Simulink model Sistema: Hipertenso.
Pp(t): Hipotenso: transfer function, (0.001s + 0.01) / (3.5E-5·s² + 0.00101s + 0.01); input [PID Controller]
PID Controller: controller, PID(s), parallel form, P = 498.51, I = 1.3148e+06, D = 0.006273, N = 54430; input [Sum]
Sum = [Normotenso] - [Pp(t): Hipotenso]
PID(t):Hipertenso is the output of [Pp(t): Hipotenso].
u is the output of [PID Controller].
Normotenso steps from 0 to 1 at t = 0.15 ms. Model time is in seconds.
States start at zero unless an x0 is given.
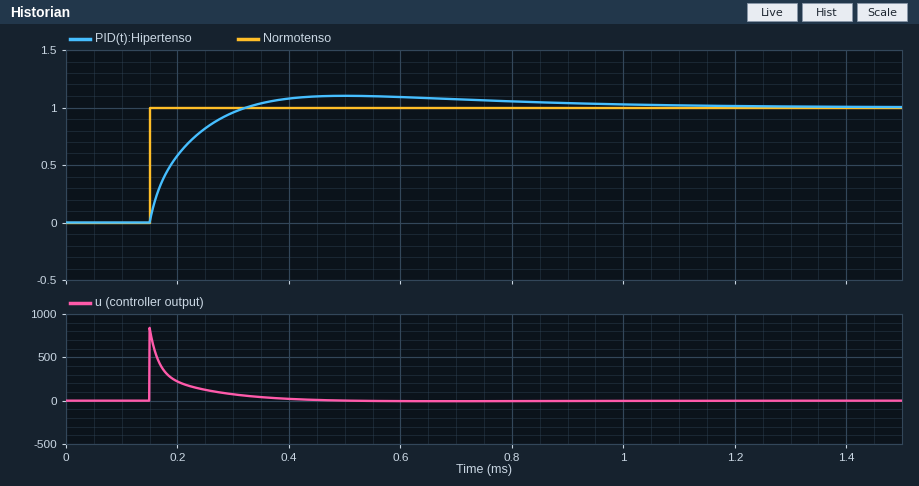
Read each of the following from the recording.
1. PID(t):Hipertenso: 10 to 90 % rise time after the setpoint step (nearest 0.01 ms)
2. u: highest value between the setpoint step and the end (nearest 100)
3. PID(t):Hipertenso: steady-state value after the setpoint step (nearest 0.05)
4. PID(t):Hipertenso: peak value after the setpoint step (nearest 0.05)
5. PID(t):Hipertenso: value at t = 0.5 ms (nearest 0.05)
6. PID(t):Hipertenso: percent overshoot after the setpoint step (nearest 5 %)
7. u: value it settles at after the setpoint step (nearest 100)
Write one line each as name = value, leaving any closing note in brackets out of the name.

PID(t):Hipertenso: 10 to 90 % rise time after the setpoint step = 0.12 ms
u: highest value between the setpoint step and the end = 800
PID(t):Hipertenso: steady-state value after the setpoint step = 1.00
PID(t):Hipertenso: peak value after the setpoint step = 1.10
PID(t):Hipertenso: value at t = 0.5 ms = 1.10
PID(t):Hipertenso: percent overshoot after the setpoint step = 10 %
u: value it settles at after the setpoint step = 0
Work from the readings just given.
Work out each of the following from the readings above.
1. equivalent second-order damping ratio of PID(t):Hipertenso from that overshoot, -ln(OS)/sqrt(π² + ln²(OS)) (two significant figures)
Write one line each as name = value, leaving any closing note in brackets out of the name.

equivalent second-order damping ratio of PID(t):Hipertenso from that overshoot, -ln(OS)/sqrt(π² + ln²(OS)) = 0.59
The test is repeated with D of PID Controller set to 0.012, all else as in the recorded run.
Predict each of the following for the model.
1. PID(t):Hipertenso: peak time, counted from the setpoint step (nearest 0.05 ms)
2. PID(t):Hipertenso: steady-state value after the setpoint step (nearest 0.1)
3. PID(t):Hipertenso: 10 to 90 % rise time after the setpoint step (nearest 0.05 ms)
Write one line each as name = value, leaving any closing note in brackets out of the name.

PID(t):Hipertenso: peak time, counted from the setpoint step = 0.40 ms
PID(t):Hipertenso: steady-state value after the setpoint step = 1.0
PID(t):Hipertenso: 10 to 90 % rise time after the setpoint step = 0.15 ms
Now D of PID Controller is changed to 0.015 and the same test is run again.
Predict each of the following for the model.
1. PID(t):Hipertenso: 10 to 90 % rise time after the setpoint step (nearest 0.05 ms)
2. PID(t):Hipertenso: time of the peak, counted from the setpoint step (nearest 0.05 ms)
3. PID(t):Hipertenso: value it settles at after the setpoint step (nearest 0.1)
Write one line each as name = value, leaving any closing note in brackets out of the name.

PID(t):Hipertenso: 10 to 90 % rise time after the setpoint step = 0.15 ms
PID(t):Hipertenso: time of the peak, counted from the setpoint step = 0.40 ms
PID(t):Hipertenso: value it settles at after the setpoint step = 1.0
